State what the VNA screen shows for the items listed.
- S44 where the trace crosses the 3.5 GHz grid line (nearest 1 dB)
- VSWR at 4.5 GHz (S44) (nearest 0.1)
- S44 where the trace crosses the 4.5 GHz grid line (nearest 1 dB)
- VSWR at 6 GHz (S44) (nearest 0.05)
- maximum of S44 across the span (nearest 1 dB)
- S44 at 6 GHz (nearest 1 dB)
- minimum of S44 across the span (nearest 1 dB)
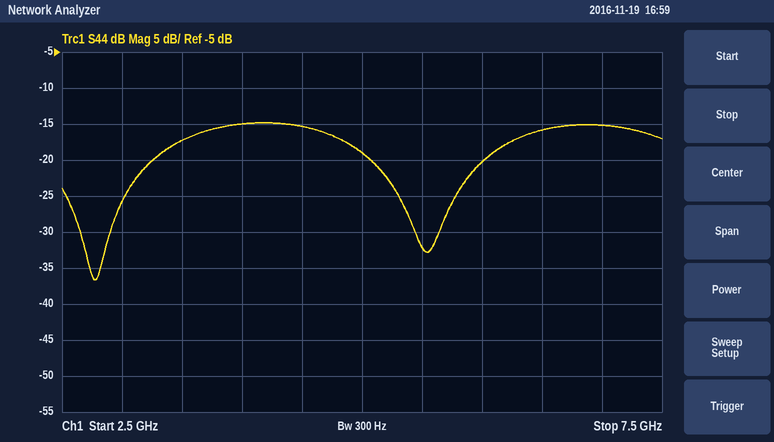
-17 dB
1.4
-15 dB
1.20
-15 dB
-20 dB
-37 dB
